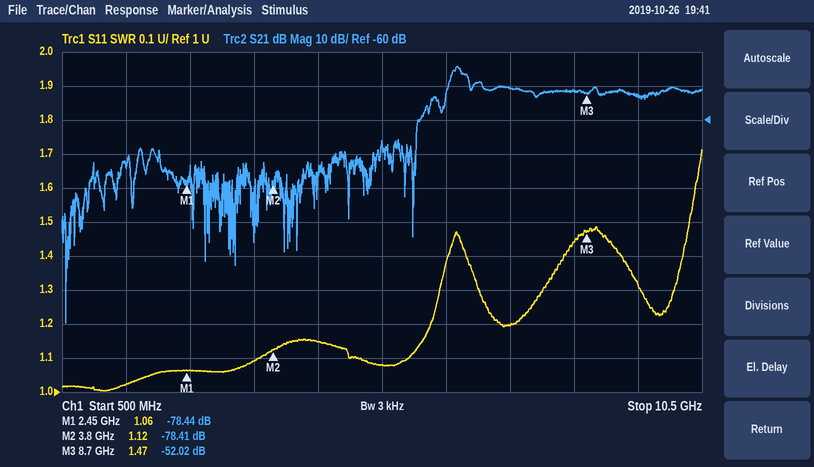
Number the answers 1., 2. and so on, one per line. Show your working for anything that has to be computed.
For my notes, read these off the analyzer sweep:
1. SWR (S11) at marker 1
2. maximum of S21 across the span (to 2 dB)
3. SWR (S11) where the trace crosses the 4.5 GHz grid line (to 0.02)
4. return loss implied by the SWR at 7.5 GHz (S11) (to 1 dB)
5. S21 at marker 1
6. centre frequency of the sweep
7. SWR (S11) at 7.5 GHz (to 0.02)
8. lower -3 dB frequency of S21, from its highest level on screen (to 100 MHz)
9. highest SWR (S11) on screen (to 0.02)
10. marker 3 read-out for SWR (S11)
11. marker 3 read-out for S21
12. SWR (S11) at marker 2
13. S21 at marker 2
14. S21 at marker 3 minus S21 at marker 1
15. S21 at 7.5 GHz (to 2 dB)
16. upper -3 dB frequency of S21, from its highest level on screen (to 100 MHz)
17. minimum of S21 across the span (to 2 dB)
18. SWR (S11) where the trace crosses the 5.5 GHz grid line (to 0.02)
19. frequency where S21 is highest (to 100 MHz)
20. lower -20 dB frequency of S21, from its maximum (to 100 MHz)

1. 1.06
2. -44 dB
3. 1.14
4. −20 log10((1.2 − 1)/(1.2 + 1)) ≈ 21 dB
5. -78.44 dB
6. 5.5 GHz
7. 1.20
8. 6.6 GHz
9. 1.72
10. 1.47
11. -52.02 dB
12. 1.12
13. -78.41 dB
14. -52.02 − (-78.44) = 26.42 dB
15. -50 dB
16. 6.8 GHz
17. -120 dB
18. 1.08
19. 6.7 GHz
20. 6.0 GHz
